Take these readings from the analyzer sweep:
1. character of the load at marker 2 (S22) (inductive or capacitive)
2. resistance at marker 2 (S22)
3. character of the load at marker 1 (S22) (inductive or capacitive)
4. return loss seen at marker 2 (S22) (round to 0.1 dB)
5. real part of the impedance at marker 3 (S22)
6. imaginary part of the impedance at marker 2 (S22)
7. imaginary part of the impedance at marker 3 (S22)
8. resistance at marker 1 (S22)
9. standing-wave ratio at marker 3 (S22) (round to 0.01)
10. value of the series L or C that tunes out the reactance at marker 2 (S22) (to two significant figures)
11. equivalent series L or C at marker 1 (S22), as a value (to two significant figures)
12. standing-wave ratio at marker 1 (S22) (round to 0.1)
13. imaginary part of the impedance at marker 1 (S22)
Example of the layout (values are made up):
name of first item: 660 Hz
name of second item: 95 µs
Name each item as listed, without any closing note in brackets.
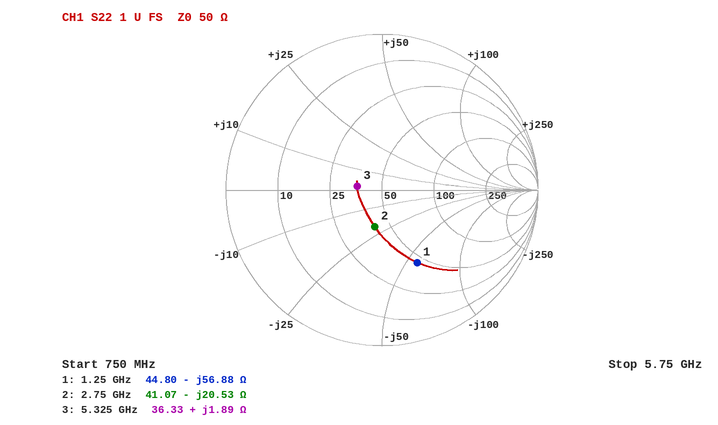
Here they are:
character of the load at marker 2 (S22): capacitive
resistance at marker 2: 41.07 Ω
character of the load at marker 1 (S22): capacitive
return loss seen at marker 2 (S22): 12.4 dB
real part of the impedance at marker 3: 36.33 Ω
imaginary part of the impedance at marker 2: -20.53 Ω
imaginary part of the impedance at marker 3: +1.89 Ω
resistance at marker 1: 44.80 Ω
standing-wave ratio at marker 3 (S22): 1.38
value of the series L or C that tunes out the reactance at marker 2 (S22): 1.2 nH
equivalent series L or C at marker 1 (S22), as a value: 2.2 pF
standing-wave ratio at marker 1 (S22): 3.1
imaginary part of the impedance at marker 1: -56.88 Ω
